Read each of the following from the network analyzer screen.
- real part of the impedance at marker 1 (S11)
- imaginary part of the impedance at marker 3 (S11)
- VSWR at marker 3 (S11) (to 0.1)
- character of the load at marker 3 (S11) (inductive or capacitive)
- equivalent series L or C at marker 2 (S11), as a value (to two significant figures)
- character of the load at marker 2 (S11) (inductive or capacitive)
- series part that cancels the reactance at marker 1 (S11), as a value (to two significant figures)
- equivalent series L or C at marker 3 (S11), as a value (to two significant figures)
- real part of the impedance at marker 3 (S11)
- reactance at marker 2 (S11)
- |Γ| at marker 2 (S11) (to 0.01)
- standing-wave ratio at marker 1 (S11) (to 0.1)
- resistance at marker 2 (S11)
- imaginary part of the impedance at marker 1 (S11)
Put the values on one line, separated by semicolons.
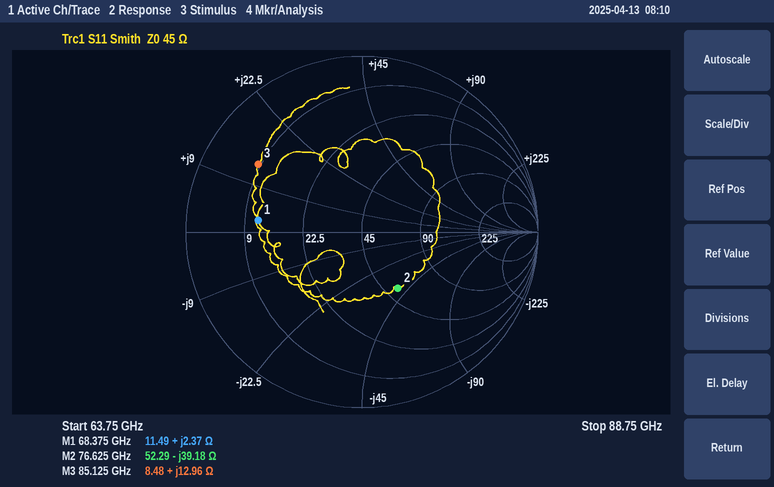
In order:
11.49 Ω; +12.96 Ω; 5.8; inductive; 53 fF; capacitive; 980 fF; 24 pH; 8.48 Ω; -39.18 Ω; 0.38; 3.9; 52.29 Ω; +2.37 Ω
